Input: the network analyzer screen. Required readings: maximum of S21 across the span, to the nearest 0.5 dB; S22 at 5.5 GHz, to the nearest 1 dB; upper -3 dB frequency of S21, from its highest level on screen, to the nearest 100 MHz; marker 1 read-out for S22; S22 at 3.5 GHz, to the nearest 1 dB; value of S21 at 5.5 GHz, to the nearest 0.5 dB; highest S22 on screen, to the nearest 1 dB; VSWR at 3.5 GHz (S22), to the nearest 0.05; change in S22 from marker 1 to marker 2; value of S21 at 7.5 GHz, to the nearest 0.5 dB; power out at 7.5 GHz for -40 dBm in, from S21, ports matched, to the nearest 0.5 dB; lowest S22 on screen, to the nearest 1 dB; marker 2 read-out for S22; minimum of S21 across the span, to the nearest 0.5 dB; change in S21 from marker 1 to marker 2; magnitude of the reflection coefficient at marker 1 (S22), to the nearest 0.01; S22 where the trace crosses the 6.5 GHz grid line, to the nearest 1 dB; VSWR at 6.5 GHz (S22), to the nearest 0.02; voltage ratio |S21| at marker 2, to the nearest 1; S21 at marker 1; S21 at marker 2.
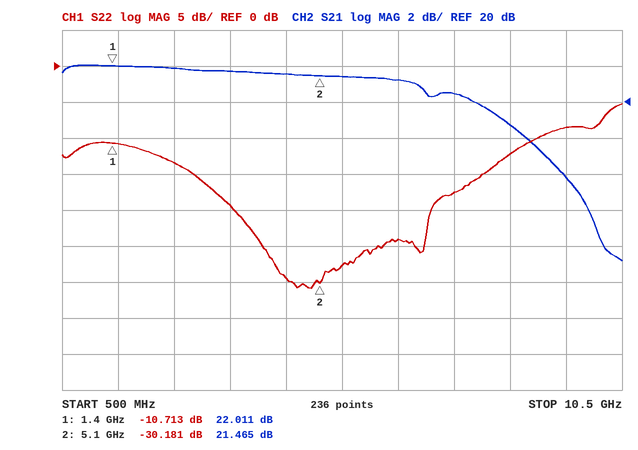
22.0 dB
-28 dB
8.4 GHz
-10.713 dB
-19 dB
21.5 dB
-5 dB
1.25
-19.468 dB
20.5 dB
-19.5 dBm
-31 dB
-30.181 dB
11.0 dB
-0.546 dB
0.29
-24 dB
1.14
12
22.011 dB
21.465 dB
